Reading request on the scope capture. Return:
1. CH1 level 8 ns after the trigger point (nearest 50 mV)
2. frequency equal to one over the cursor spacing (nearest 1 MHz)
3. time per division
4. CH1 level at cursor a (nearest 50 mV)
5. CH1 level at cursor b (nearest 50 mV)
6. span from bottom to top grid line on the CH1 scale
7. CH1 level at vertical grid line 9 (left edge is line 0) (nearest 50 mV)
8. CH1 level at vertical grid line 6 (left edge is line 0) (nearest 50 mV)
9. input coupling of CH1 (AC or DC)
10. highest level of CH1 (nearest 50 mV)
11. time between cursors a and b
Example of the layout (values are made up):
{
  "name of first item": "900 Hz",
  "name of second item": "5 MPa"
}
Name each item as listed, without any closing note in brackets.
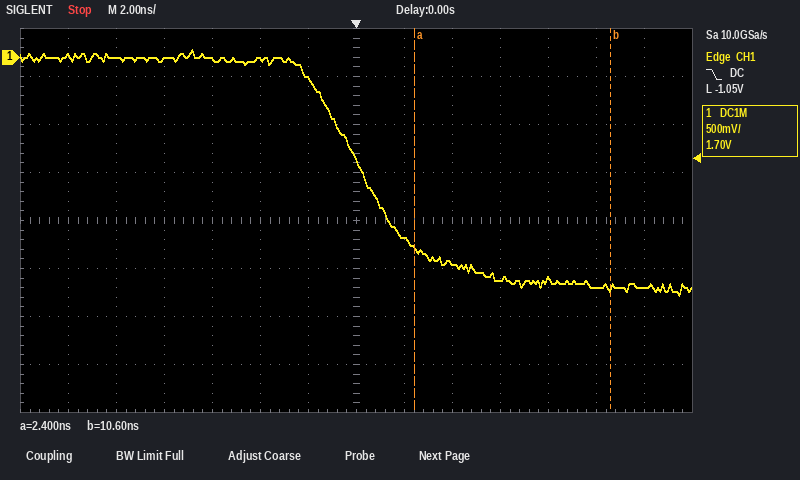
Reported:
{
  "CH1 level 8 ns after the trigger point": "-2.30 V",
  "frequency equal to one over the cursor spacing": "122 MHz",
  "time per division": "2 ns",
  "CH1 level at cursor a": "-2.00 V",
  "CH1 level at cursor b": "-2.40 V",
  "span from bottom to top grid line on the CH1 scale": "4 V",
  "CH1 level at vertical grid line 9 (left edge is line 0)": "-2.15 V",
  "CH1 level at vertical grid line 6 (left edge is line 0)": "-200 mV",
  "input coupling of CH1": "DC",
  "highest level of CH1": "100 mV",
  "time between cursors a and b": "8.2 ns"
}
